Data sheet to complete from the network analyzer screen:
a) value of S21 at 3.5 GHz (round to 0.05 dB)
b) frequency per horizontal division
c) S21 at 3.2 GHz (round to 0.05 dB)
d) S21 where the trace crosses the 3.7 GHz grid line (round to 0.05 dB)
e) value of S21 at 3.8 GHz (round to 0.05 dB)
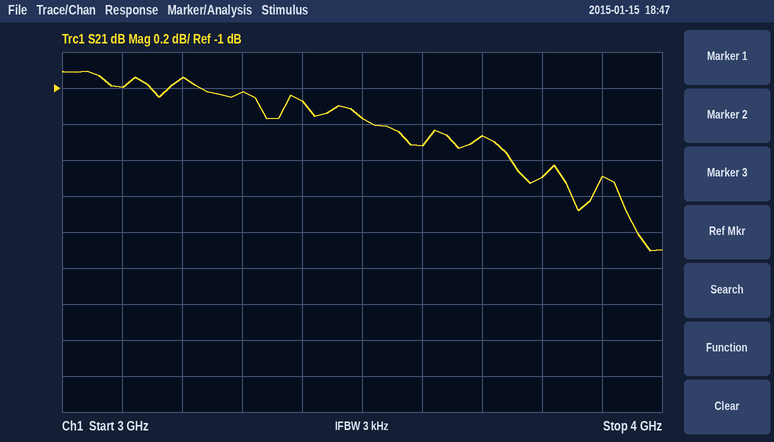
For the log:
-1.15 dB
100 MHz
-0.95 dB
-1.25 dB
-1.50 dB
